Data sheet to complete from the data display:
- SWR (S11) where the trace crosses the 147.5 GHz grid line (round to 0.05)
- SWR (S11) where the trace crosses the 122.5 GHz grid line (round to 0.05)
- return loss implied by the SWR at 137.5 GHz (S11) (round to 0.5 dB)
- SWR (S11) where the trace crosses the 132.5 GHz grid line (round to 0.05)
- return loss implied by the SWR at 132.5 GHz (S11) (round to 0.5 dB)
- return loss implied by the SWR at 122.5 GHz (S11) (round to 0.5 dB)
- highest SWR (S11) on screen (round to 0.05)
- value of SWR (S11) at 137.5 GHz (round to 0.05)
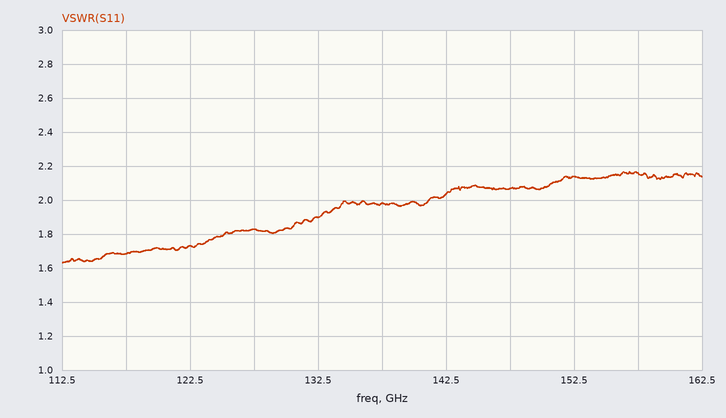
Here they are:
2.05
1.75
9.5 dB
1.90
10.0 dB
11.5 dB
2.15
2.00
